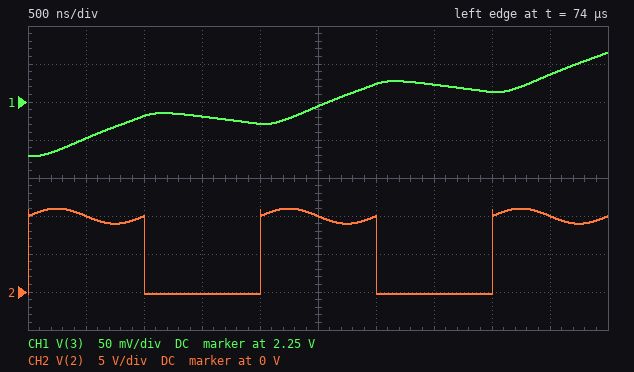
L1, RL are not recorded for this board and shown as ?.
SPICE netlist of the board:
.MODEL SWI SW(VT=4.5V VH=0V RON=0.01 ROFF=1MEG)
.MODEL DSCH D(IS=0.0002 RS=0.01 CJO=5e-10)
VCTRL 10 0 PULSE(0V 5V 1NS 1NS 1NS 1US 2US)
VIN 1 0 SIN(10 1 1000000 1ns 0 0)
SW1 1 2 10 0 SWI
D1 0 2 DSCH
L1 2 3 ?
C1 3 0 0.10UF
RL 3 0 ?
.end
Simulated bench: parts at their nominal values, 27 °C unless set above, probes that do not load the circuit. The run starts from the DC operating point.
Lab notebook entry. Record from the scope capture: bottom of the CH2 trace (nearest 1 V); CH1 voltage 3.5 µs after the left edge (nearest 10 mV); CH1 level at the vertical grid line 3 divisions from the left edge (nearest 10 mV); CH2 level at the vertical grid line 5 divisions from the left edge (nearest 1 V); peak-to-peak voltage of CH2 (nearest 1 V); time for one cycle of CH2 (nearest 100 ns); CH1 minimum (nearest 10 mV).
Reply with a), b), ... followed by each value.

a) 0 V
b) 2.27 V
c) 2.23 V
d) 10 V
e) 11 V
f) 2.0 µs
g) 2.18 V
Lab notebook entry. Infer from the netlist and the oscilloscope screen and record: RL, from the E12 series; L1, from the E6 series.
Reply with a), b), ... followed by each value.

a) 1.2 Ω
b) 150 µH
